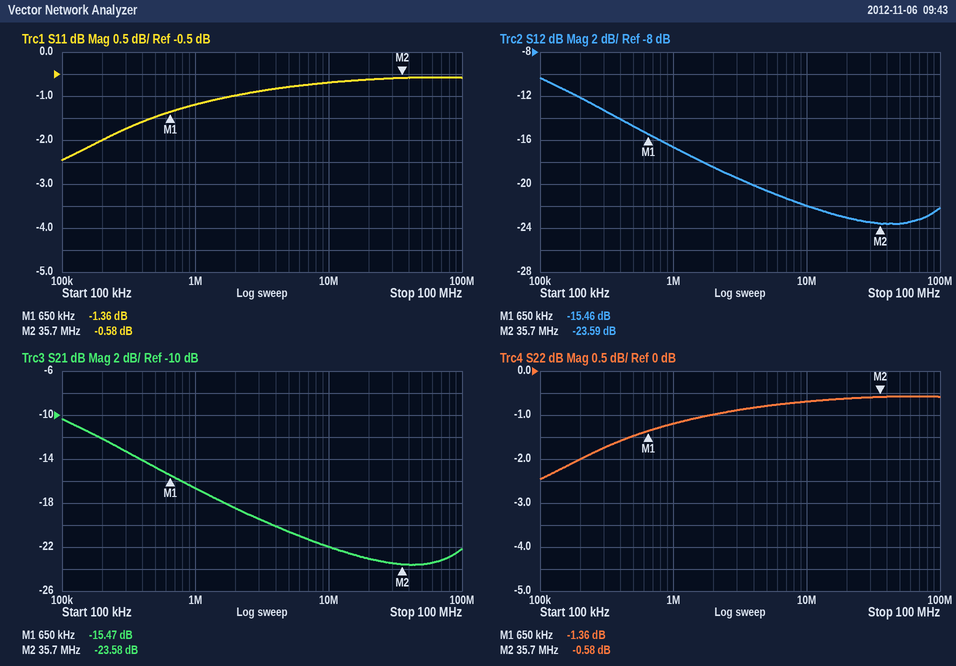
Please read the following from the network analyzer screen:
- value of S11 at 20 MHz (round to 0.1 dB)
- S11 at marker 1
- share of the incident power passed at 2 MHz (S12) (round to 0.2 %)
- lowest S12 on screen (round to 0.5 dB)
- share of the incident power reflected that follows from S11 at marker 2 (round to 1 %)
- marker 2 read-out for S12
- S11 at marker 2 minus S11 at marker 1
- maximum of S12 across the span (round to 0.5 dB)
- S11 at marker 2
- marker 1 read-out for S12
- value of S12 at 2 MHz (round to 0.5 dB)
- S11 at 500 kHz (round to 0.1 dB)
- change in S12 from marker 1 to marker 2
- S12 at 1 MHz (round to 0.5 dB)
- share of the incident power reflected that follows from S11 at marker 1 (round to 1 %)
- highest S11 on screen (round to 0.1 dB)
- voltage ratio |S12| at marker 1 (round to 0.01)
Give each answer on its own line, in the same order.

-0.6 dB
-1.36 dB
1.4 %
-23.5 dB
87 %
-23.59 dB
0.78 dB
-10.5 dB
-0.58 dB
-15.46 dB
-18.5 dB
-1.5 dB
-8.13 dB
-16.5 dB
73 %
-0.6 dB
0.17
